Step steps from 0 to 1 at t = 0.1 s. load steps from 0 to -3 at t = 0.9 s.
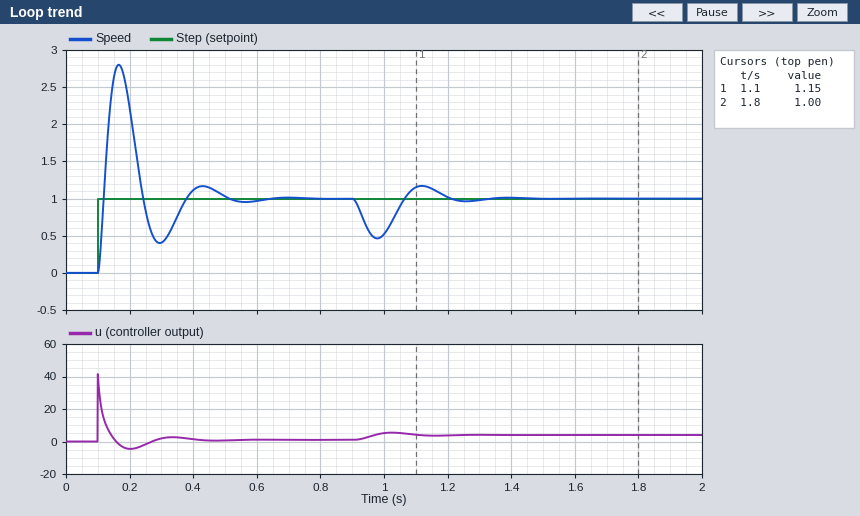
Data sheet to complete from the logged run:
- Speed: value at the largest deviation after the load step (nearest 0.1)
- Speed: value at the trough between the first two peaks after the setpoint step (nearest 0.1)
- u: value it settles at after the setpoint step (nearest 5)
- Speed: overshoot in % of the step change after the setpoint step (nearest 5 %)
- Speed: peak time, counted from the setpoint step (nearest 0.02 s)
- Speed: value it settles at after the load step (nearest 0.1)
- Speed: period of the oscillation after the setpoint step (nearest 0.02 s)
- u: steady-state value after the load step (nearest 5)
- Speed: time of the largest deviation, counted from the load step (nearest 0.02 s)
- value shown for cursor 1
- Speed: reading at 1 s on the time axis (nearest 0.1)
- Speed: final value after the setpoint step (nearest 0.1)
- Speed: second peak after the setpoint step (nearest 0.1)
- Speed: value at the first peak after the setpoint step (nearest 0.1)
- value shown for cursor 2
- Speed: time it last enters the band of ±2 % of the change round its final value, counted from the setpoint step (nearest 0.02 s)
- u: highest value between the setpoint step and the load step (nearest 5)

0.5
0.4
0
180 %
0.06 s
1.0
0.26 s
5
0.08 s
1.15
0.5
1.0
1.2
2.8
1.00
0.52 s
40
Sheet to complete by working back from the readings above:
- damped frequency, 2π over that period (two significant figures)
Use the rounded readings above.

24 rad/s
